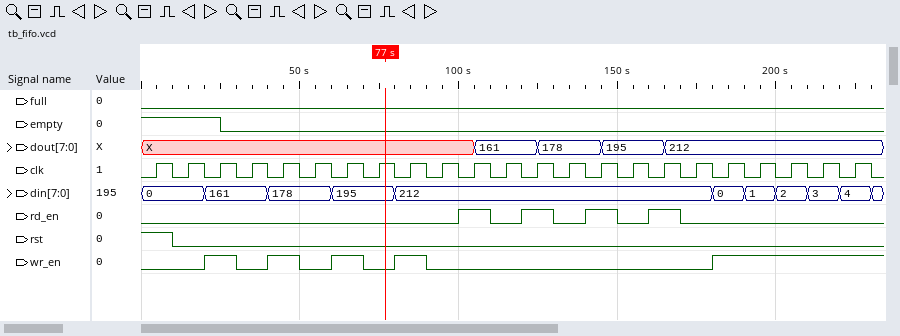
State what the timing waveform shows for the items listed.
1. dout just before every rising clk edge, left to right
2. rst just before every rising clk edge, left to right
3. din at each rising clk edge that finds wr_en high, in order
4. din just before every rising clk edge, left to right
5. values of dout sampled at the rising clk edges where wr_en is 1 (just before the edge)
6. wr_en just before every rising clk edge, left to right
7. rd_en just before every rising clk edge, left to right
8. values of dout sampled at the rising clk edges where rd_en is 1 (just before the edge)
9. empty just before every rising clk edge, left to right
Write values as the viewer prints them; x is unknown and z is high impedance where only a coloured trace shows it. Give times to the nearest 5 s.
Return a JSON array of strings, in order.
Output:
["X, X, X, X, X, X, X, X, X, X, X, 161, 161, 178, 178, 195, 195, 212, 212, 212, 212, 212, 212", "1 0 0 0 0 0 0 0 0 0 0 0 0 0 0 0 0 0 0 0 0 0 0", "161, 178, 195, 212, 0, 1, 2, 3, 4", "0, 0, 161, 161, 178, 178, 195, 195, 212, 212, 212, 212, 212, 212, 212, 212, 212, 212, 0, 1, 2, 3, 4", "X, X, X, X, 212, 212, 212, 212, 212", "0 0 1 0 1 0 1 0 1 0 0 0 0 0 0 0 0 0 1 1 1 1 1", "0 0 0 0 0 0 0 0 0 0 1 0 1 0 1 0 1 0 0 0 0 0 0", "X, 161, 178, 195", "1 1 1 0 0 0 0 0 0 0 0 0 0 0 0 0 0 0 0 0 0 0 0"]
